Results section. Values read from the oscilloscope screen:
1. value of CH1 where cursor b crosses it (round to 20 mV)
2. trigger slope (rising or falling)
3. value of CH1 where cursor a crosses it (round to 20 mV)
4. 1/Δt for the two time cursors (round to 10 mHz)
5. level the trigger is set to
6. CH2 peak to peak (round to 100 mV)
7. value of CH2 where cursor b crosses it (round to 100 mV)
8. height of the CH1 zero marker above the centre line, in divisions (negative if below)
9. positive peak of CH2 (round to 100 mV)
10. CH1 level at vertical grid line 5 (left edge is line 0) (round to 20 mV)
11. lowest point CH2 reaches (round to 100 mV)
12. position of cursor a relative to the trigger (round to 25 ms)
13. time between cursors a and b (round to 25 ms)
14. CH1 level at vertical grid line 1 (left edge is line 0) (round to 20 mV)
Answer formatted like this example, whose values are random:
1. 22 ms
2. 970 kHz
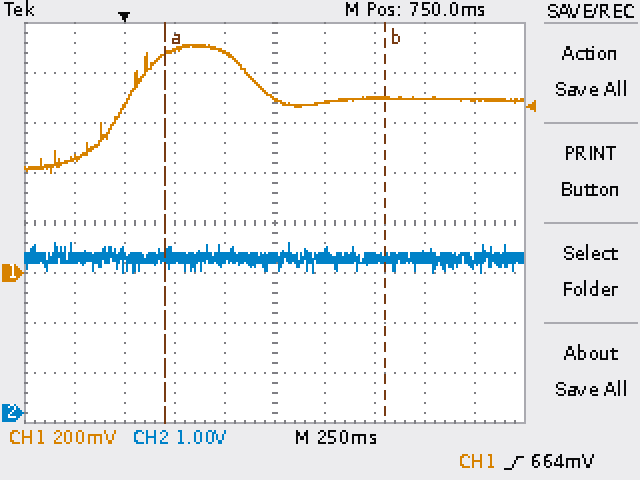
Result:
1. 700 mV
2. rising
3. 880 mV
4. 910 mHz
5. 664 mV
6. 600 mV
7. 3.1 V
8. -1.0 div
9. 3.4 V
10. 700 mV
11. 2.8 V
12. +200 ms
13. 1.100 s
14. 460 mV
